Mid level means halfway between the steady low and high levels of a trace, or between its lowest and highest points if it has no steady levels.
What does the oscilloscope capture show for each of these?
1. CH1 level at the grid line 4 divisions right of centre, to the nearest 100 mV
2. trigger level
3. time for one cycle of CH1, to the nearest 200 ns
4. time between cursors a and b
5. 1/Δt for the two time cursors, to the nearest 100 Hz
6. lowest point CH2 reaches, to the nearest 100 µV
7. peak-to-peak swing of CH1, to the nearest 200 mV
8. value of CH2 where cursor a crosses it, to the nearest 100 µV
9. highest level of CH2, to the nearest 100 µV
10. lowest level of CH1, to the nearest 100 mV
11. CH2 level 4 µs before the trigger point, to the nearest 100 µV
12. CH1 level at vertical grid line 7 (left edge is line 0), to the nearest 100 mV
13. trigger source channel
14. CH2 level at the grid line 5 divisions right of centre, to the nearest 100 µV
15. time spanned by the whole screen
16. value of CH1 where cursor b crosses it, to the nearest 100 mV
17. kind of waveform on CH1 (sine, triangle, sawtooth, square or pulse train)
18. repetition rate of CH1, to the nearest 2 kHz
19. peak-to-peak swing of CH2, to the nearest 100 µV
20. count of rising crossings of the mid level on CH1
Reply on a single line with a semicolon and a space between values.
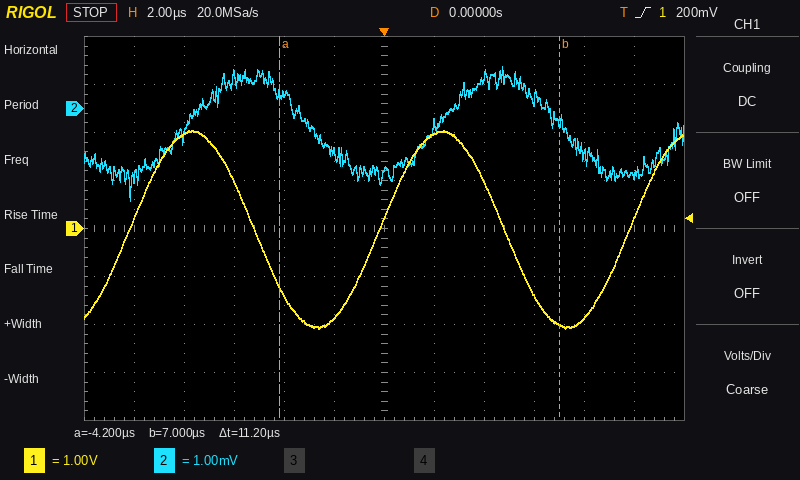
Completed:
-1.9 V; 200 mV; 10.0 µs; 11.2 µs; 89.3 kHz; -1.9 mV; 4.2 V; 300 µV; 900 µV; -2.1 V; 300 µV; 2.0 V; CH1; -1.4 mV; 24 µs; -2.0 V; sine; 100 kHz; 2.8 mV; 3
